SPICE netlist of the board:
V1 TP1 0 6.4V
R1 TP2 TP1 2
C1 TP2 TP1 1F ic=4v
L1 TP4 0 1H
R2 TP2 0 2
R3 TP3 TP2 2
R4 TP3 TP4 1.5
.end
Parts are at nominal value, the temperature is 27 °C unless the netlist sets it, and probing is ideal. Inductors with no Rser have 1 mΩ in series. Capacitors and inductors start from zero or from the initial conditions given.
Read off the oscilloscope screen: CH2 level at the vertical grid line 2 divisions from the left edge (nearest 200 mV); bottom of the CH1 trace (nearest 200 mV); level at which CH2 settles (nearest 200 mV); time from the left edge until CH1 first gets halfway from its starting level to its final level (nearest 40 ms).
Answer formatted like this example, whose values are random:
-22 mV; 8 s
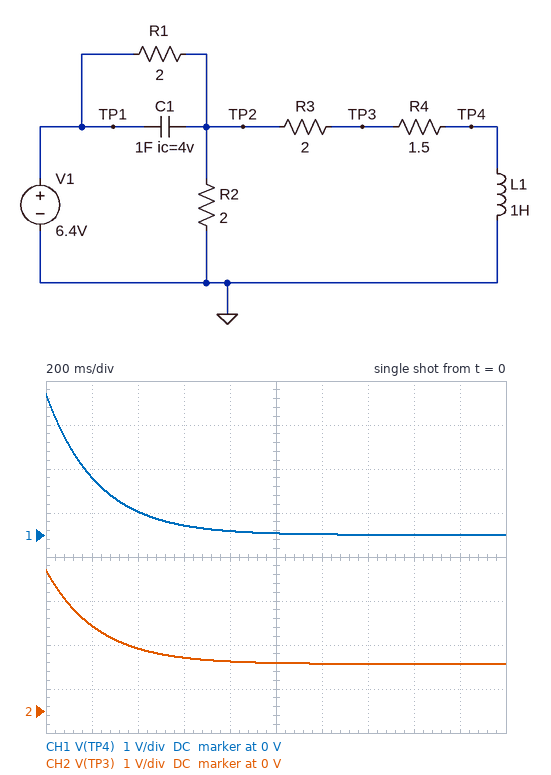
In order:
1.4 V; 0 V; 1.0 V; 160 ms
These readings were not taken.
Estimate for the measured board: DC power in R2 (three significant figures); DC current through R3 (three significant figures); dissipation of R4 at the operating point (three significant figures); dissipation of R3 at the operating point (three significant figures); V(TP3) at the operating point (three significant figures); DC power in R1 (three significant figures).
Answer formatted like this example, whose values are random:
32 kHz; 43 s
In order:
3.10 W; 711 mA; 758 mW; 1.01 W; 1.07 V; 7.65 W
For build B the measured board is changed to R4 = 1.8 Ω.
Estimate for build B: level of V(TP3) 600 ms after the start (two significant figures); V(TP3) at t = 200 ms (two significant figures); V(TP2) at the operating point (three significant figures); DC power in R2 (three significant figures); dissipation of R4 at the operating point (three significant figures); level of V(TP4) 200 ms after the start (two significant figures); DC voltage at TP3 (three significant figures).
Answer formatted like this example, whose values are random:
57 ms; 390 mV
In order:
1.3 V; 2.0 V; 2.53 V; 3.21 W; 800 mW; 1.2 V; 1.20 V
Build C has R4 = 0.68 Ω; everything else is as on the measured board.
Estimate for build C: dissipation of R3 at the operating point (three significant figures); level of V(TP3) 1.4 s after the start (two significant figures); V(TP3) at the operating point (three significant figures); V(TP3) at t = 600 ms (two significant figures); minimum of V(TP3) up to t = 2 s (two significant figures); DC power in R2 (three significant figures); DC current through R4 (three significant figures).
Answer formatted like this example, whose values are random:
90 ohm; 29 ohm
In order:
1.51 W; 610 mV; 592 mV; 880 mV; 590 mV; 2.72 W; 869 mA
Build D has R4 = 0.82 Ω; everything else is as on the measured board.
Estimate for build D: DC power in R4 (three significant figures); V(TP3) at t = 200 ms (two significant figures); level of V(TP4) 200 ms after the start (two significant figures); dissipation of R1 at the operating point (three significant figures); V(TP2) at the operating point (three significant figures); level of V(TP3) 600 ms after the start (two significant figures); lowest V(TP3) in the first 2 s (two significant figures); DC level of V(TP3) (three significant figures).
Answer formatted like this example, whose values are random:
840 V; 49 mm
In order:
575 mW; 1.9 V; 1.5 V; 8.15 W; 2.36 V; 940 mV; 690 mV; 688 mV
